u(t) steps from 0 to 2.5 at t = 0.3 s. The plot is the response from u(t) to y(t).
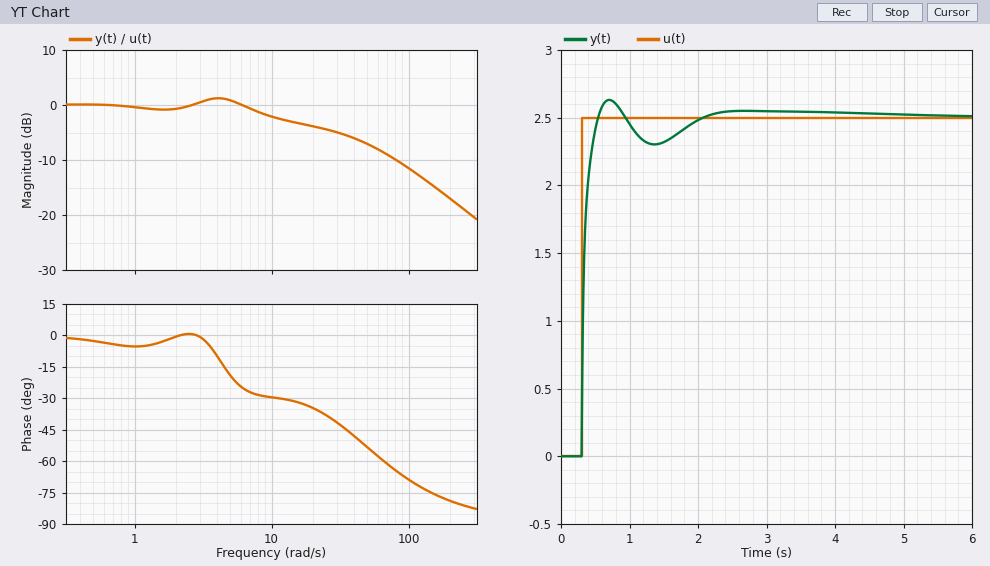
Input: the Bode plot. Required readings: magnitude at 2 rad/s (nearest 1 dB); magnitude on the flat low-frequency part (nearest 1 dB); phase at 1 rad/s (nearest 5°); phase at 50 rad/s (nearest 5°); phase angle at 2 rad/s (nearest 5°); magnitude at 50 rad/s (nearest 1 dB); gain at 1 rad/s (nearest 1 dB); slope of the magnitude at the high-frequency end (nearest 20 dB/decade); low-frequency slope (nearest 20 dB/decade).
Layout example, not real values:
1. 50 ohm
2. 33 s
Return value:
1. -1 dB
2. 0 dB
3. -5°
4. -55°
5. 0°
6. -7 dB
7. 0 dB
8. -20 dB/decade
9. 0 dB/decade
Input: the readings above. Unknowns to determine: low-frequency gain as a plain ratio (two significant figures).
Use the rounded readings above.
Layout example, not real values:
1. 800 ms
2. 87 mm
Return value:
1. 1.0
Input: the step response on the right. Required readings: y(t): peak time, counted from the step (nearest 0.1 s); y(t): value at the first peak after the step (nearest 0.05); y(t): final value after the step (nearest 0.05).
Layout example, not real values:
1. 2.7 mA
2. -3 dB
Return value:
1. 0.4 s
2. 2.65
3. 2.50
